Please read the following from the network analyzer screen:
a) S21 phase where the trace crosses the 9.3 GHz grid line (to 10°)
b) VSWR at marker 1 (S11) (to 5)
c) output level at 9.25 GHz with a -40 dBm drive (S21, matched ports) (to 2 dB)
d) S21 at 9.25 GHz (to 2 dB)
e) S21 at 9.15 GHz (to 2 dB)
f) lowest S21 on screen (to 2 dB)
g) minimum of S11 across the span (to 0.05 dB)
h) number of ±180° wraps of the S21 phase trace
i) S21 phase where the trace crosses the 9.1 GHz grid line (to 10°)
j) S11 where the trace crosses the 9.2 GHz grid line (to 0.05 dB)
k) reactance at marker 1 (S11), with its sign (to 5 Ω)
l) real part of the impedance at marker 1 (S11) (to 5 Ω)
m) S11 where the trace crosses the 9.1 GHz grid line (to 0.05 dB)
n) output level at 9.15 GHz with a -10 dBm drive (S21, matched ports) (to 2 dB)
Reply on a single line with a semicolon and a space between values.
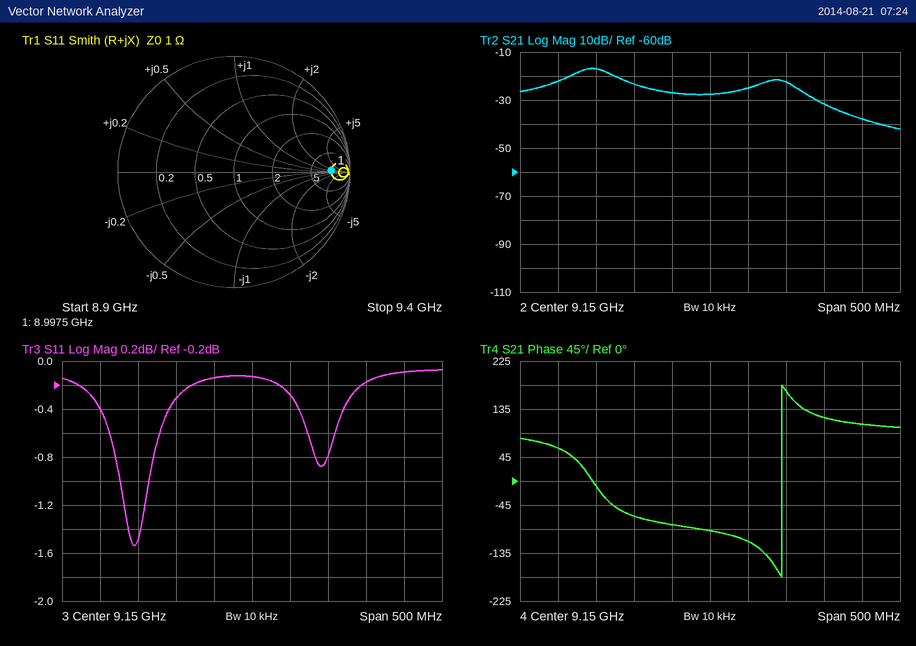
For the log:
120°; 10; -62 dBm; -22 dB; -28 dB; -42 dB; -1.55 dB; 1; -80°; -0.30 dB; 0 Ω; 10 Ω; -0.15 dB; -38 dBm
